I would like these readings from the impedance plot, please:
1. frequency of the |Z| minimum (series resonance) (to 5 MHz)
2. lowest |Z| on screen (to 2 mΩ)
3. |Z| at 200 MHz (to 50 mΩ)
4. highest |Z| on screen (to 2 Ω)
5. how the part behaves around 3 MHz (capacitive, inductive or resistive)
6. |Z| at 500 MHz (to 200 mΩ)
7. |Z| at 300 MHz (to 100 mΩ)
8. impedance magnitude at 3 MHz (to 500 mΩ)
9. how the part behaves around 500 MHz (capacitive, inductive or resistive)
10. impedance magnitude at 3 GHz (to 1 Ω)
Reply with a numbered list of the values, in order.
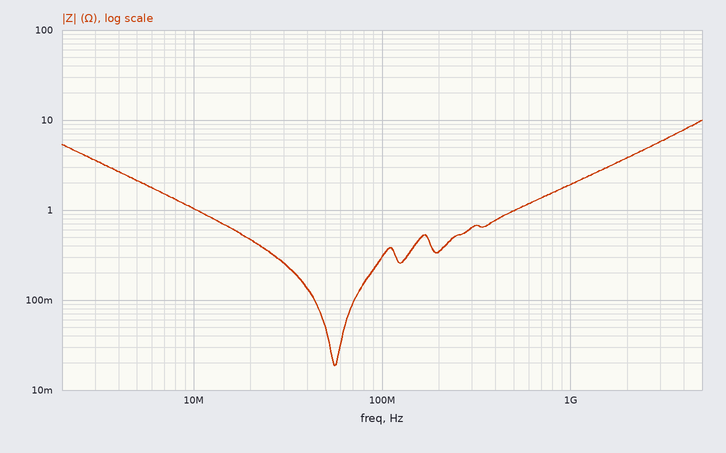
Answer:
1. 55 MHz
2. 18 mΩ
3. 350 mΩ
4. 10 Ω
5. capacitive
6. 1.0 Ω
7. 600 mΩ
8. 3.5 Ω
9. inductive
10. 6 Ω
